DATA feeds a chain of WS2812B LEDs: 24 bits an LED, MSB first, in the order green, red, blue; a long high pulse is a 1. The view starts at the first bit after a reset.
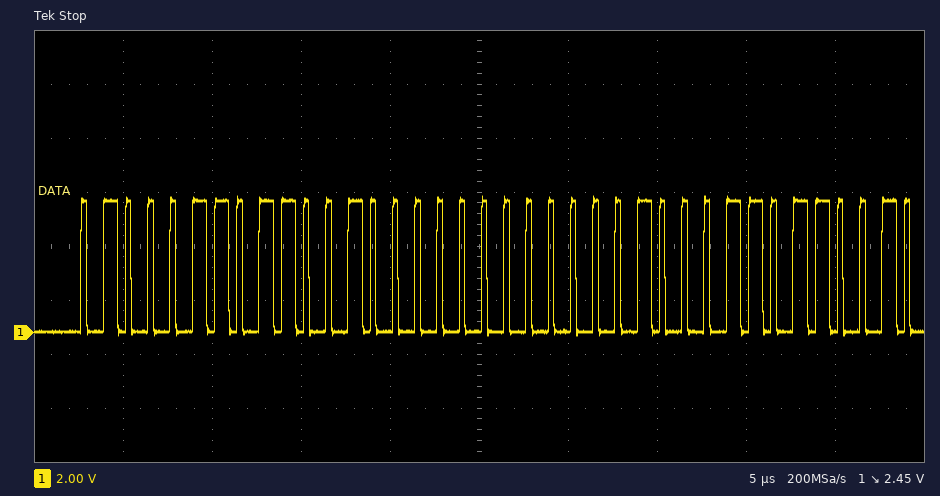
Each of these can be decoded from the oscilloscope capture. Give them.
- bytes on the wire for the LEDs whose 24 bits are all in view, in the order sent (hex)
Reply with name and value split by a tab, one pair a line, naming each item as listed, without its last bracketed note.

bytes on the wire for the LEDs whose 24 bits are all in view, in the order sent	46 C8 00
